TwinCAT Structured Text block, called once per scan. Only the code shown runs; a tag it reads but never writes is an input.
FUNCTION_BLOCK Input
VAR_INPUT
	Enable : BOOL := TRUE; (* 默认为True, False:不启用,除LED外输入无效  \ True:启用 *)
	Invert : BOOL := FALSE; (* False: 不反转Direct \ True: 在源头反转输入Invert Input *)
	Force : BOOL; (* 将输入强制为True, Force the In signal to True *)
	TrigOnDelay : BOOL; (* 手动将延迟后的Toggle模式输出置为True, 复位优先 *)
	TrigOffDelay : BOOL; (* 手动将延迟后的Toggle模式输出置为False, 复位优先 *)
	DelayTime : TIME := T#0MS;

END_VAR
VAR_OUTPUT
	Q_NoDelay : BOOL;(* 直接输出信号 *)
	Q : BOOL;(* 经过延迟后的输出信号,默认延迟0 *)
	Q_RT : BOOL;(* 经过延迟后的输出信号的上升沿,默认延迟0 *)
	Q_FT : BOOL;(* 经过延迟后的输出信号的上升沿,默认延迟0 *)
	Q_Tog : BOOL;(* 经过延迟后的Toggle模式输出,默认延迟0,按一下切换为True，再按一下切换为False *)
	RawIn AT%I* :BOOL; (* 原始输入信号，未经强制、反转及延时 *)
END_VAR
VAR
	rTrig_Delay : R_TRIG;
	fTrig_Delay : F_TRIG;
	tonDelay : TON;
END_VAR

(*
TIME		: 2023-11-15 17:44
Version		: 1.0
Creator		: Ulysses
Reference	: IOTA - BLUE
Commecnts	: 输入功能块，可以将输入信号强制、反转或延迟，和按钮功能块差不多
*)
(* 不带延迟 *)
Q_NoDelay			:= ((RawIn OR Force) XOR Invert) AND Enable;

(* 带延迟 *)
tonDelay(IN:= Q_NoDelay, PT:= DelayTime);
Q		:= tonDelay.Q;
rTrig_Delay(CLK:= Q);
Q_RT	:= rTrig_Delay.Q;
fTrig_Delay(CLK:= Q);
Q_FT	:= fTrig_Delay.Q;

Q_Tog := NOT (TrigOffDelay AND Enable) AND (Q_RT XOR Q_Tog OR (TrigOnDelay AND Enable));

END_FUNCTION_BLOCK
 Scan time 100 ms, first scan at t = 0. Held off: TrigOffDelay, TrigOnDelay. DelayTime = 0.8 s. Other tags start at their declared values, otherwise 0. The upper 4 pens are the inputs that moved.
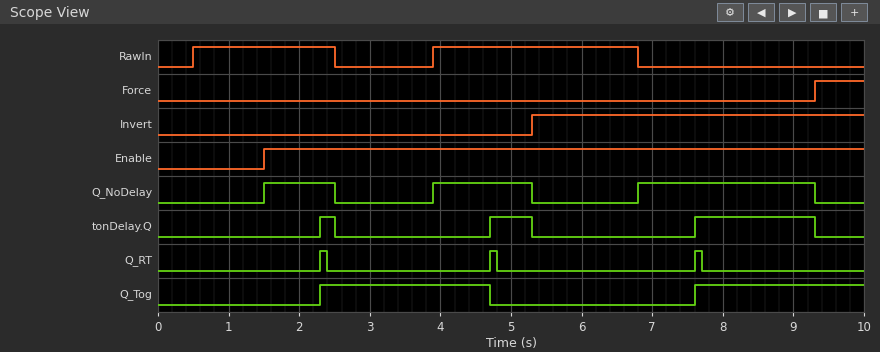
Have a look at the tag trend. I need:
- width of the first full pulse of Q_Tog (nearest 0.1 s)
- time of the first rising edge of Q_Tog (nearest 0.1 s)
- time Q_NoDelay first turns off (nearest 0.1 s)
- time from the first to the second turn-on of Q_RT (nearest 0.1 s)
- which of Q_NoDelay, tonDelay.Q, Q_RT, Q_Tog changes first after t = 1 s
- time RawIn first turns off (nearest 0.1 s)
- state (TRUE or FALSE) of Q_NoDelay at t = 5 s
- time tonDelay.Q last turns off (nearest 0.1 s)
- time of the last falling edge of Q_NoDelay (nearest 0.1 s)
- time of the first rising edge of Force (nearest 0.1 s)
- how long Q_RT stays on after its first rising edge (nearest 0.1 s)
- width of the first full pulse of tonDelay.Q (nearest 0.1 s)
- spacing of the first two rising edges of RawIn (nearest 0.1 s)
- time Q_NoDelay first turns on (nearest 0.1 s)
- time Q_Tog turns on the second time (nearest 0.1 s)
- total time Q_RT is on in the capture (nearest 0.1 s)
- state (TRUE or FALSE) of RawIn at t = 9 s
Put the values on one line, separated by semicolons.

2.4 s; 2.3 s; 2.5 s; 2.4 s; Q_NoDelay; 2.5 s; TRUE; 9.3 s; 9.3 s; 9.3 s; 0.1 s; 0.2 s; 3.4 s; 1.5 s; 7.6 s; 0.3 s; FALSE
